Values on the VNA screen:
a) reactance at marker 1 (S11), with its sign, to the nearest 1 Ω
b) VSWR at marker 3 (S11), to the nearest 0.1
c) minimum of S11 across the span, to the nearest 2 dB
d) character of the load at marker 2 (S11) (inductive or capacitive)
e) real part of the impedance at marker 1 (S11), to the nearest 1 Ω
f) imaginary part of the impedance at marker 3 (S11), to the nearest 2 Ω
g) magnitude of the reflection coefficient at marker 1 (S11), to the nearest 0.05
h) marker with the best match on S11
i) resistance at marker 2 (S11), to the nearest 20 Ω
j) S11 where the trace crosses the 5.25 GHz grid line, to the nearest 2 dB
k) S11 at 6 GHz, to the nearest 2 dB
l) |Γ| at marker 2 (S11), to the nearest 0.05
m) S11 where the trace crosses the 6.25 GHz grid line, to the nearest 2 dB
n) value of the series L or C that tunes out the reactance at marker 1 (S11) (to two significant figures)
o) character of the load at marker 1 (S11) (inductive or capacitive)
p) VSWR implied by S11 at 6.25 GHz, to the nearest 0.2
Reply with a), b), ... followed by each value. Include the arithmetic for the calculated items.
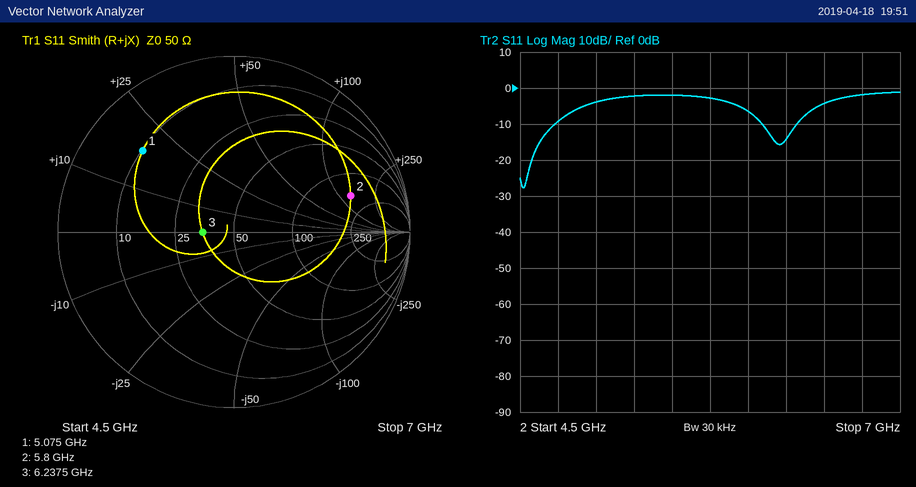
a) +18 Ω
b) 1.4
c) -28 dB
d) inductive
e) 10 Ω
f) 0 Ω
g) 0.70
h) marker 3
i) 160 Ω
j) -2 dB
k) -6 dB
l) 0.70
m) -14 dB
n) C = 1/(2π × 5.075 GHz × 18 Ω) ≈ 1.7 pF
o) inductive
p) |Γ| = 10^(-14/20) = 0.1995; VSWR = (1 + 0.1995)/(1 − 0.1995) ≈ 1.50, so 1.4 to the nearest 0.2
